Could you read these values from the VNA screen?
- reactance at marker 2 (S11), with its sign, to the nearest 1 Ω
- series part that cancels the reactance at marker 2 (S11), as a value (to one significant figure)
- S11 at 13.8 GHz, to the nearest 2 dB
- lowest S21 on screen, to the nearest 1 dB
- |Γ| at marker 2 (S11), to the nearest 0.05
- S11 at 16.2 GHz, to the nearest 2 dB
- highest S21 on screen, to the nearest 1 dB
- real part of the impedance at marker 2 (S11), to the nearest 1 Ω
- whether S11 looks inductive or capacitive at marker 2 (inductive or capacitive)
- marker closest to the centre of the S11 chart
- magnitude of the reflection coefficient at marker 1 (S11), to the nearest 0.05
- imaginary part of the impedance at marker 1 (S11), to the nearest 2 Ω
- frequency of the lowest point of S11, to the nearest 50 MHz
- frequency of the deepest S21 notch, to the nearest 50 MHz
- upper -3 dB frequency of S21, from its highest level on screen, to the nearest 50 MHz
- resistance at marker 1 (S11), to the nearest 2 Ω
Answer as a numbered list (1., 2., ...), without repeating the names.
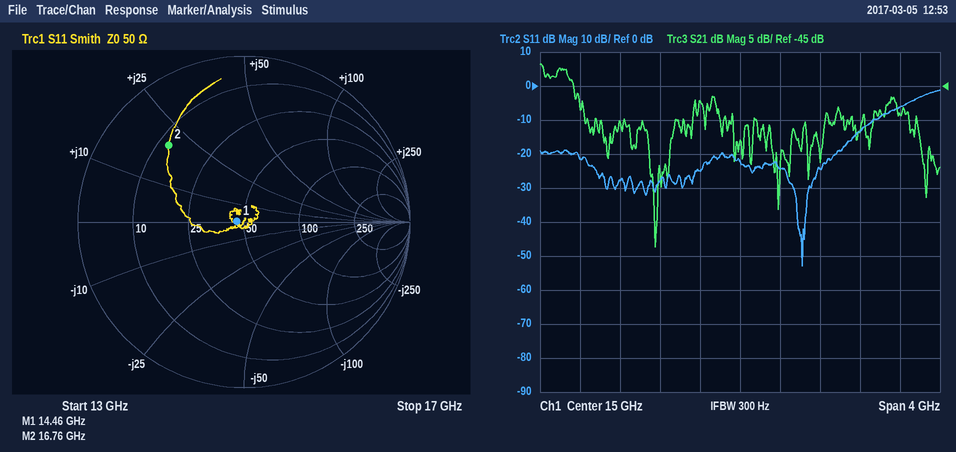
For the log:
1. +20 Ω
2. 500 fF
3. -28 dB
4. -69 dB
5. 0.65
6. -14 dB
7. -42 dB
8. 12 Ω
9. inductive
10. marker 1
11. 0.05
12. 0 Ω
13. 15.60 GHz
14. 14.15 GHz
15. 13.35 GHz
16. 46 Ω
